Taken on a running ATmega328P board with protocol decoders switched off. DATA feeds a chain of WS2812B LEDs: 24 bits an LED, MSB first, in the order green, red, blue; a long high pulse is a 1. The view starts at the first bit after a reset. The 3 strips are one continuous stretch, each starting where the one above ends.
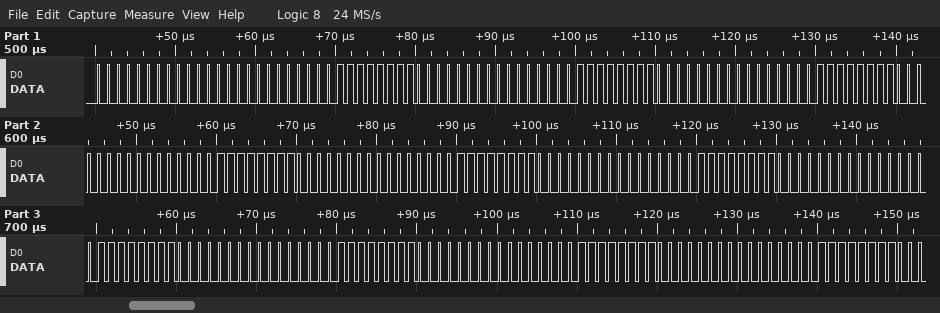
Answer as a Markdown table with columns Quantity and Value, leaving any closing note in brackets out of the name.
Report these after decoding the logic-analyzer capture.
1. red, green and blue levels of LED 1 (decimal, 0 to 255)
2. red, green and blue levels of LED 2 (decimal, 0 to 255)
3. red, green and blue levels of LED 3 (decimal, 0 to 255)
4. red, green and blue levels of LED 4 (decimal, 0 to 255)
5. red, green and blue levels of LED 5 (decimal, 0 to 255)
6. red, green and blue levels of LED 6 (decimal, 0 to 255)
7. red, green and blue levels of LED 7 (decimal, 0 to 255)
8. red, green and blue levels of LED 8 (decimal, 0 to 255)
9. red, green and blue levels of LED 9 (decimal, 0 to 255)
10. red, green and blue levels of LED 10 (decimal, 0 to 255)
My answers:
| Quantity | Value |
|---|---|
| red, green and blue levels of LED 1 | 0, 0, 0 |
| red, green and blue levels of LED 2 | 0, 255, 0 |
| red, green and blue levels of LED 3 | 0, 255, 0 |
| red, green and blue levels of LED 4 | 0, 255, 0 |
| red, green and blue levels of LED 5 | 0, 255, 0 |
| red, green and blue levels of LED 6 | 0, 255, 0 |
| red, green and blue levels of LED 7 | 0, 255, 0 |
| red, green and blue levels of LED 8 | 0, 255, 0 |
| red, green and blue levels of LED 9 | 0, 255, 0 |
| red, green and blue levels of LED 10 | 0, 255, 0 |
